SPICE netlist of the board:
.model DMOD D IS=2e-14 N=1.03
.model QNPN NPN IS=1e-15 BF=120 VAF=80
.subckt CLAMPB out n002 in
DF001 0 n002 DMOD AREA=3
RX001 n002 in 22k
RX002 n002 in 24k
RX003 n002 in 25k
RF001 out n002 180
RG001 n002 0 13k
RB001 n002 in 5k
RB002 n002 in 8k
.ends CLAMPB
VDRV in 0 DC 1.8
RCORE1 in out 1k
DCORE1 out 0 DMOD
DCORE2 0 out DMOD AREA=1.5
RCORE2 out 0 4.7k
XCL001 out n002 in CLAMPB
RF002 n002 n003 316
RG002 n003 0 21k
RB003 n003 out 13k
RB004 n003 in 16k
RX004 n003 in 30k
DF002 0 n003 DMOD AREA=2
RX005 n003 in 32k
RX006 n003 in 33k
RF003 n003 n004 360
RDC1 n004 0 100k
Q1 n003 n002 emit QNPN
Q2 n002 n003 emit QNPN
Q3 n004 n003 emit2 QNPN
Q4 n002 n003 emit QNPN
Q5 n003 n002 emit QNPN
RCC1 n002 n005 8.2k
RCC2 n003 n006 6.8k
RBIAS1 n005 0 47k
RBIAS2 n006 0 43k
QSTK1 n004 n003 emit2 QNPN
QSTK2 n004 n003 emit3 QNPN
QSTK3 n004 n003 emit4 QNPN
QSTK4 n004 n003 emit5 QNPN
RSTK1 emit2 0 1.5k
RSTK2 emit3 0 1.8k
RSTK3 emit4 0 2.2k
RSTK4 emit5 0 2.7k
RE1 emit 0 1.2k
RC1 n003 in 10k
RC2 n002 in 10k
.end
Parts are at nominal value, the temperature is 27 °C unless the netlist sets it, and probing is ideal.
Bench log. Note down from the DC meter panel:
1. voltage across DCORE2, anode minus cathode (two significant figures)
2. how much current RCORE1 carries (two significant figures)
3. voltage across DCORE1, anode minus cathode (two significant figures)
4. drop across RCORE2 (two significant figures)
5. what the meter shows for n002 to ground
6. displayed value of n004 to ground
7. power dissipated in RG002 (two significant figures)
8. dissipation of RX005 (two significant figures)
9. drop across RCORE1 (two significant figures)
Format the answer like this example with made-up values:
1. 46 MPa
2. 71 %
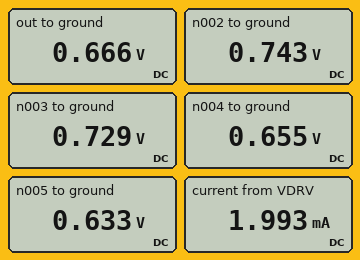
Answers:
1. -670 mV
2. 1.1 mA
3. 670 mV
4. 670 mV
5. 0.743 V
6. 0.655 V
7. 25 µW
8. 36 µW
9. 1.1 V
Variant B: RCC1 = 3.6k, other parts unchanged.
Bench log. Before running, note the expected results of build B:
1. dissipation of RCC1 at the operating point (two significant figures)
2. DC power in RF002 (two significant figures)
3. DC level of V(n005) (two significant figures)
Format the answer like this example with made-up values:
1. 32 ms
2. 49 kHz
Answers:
1. 780 nW
2. 670 nW
3. 690 mV
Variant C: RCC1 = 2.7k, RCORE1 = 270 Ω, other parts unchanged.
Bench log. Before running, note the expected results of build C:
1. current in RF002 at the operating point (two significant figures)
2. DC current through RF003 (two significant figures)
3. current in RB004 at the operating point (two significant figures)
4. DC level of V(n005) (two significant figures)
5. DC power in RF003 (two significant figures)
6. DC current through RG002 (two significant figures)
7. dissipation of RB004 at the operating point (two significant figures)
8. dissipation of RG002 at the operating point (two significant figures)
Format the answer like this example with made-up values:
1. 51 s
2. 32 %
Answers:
1. 82 µA
2. 220 µA
3. 66 µA
4. 720 mV
5. 17 µW
6. 35 µA
7. 70 µW
8. 26 µW
